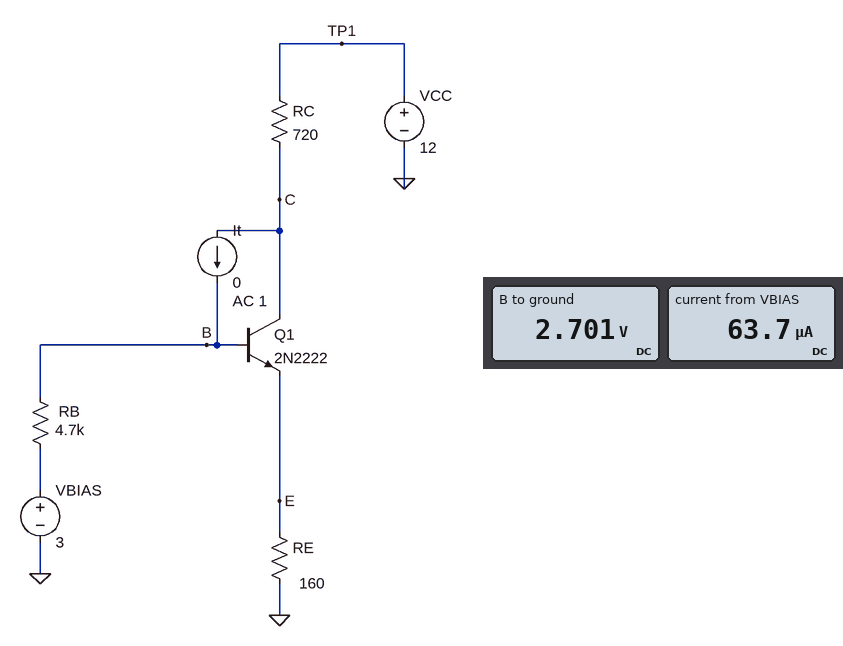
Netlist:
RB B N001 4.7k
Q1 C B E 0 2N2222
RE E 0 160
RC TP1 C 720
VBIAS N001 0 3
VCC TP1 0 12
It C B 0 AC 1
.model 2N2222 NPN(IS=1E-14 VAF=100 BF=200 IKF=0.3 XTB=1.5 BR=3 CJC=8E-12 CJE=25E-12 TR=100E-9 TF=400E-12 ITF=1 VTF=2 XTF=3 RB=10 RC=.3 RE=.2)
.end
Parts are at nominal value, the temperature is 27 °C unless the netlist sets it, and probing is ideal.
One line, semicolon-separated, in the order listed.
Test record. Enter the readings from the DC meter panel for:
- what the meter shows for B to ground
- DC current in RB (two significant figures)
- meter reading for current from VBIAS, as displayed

2.701 V; 64 µA; 63.7 µA
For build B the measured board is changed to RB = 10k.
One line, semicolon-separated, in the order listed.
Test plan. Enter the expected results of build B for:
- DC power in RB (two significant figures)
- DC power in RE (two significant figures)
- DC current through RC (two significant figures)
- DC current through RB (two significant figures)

30 µW; 19 mW; 11 mA; 55 µA
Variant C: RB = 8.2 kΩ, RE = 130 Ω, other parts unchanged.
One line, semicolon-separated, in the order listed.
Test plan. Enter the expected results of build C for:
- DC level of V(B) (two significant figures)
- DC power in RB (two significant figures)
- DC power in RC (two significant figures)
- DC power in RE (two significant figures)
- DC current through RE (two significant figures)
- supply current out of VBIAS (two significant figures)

2.4 V; 38 µW; 120 mW; 23 mW; 13 mA; 68 µA
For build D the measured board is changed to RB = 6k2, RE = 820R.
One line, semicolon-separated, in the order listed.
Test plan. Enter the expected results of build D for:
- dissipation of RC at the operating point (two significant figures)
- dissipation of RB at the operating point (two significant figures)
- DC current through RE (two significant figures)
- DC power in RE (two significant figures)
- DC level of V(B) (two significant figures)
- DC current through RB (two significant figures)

5.3 mW; 1.0 µW; 2.7 mA; 6.1 mW; 2.9 V; 13 µA
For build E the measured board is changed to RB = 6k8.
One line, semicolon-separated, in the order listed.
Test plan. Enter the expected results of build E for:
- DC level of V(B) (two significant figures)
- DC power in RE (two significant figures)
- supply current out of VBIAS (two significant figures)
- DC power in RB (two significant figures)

2.6 V; 22 mW; 60 µA; 24 µW
